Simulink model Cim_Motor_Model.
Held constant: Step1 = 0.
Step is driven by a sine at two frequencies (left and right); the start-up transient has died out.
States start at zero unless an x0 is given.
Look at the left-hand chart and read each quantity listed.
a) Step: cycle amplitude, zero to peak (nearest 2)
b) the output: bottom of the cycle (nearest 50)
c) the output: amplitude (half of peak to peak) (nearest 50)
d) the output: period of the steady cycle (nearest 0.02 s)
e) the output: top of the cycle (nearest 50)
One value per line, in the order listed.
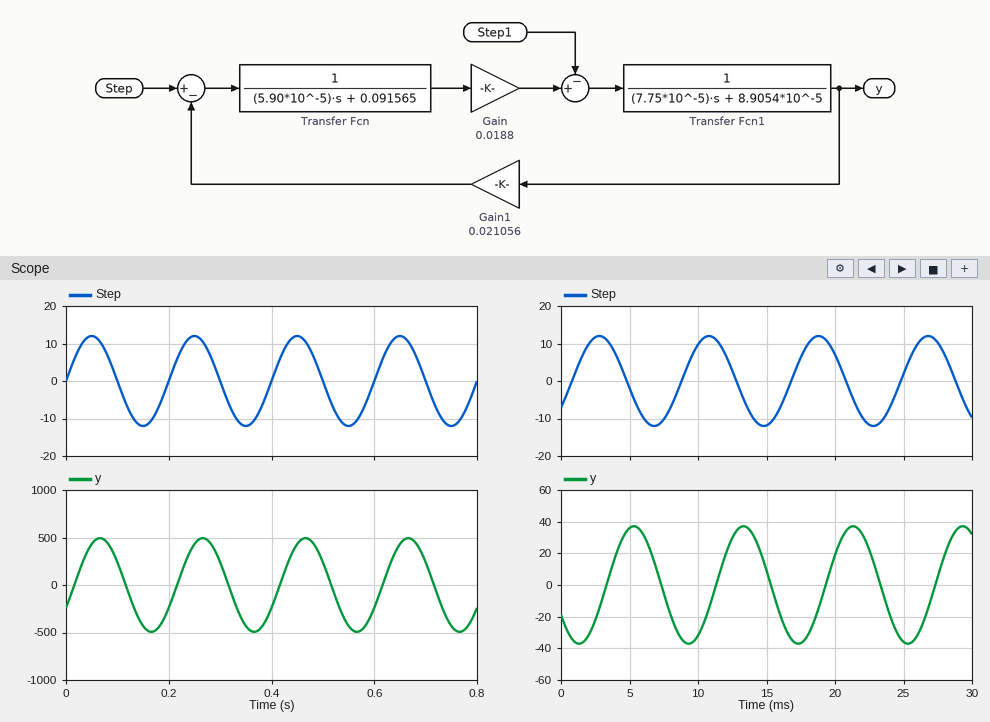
12
-500
500
0.20 s
500
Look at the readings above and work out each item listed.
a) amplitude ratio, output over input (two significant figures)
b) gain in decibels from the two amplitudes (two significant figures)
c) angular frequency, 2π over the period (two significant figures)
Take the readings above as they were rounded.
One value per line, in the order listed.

42
32 dB
31 rad/s
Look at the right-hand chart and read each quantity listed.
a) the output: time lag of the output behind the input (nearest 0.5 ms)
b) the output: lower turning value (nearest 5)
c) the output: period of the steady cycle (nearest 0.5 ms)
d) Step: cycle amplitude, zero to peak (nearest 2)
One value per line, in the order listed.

2.5 ms
-35
8.0 ms
12
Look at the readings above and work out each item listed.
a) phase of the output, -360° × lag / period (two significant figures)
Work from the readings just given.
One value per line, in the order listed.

-110°
